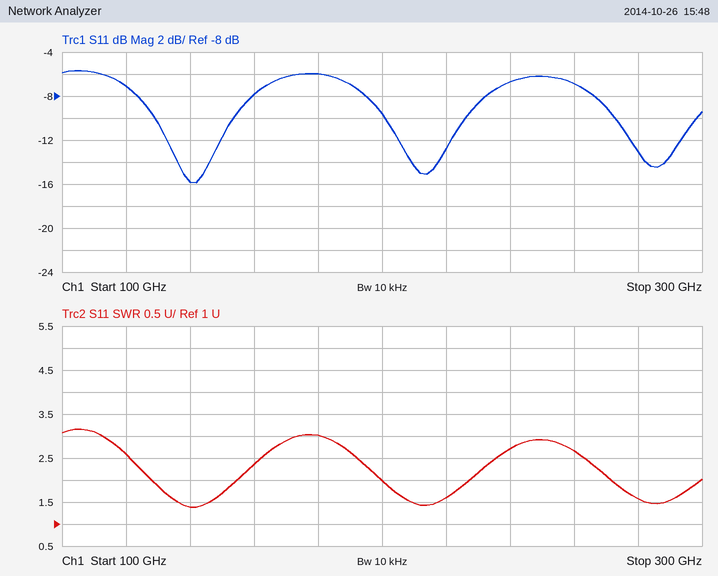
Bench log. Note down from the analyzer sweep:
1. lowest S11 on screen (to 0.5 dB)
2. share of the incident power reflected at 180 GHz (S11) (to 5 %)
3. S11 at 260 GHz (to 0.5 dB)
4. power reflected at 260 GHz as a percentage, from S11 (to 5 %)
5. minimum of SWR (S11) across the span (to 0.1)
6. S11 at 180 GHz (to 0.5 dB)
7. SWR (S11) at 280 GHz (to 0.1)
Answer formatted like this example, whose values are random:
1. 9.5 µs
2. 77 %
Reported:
1. -16.0 dB
2. 25 %
3. -7.0 dB
4. 20 %
5. 1.4
6. -6.0 dB
7. 1.6
